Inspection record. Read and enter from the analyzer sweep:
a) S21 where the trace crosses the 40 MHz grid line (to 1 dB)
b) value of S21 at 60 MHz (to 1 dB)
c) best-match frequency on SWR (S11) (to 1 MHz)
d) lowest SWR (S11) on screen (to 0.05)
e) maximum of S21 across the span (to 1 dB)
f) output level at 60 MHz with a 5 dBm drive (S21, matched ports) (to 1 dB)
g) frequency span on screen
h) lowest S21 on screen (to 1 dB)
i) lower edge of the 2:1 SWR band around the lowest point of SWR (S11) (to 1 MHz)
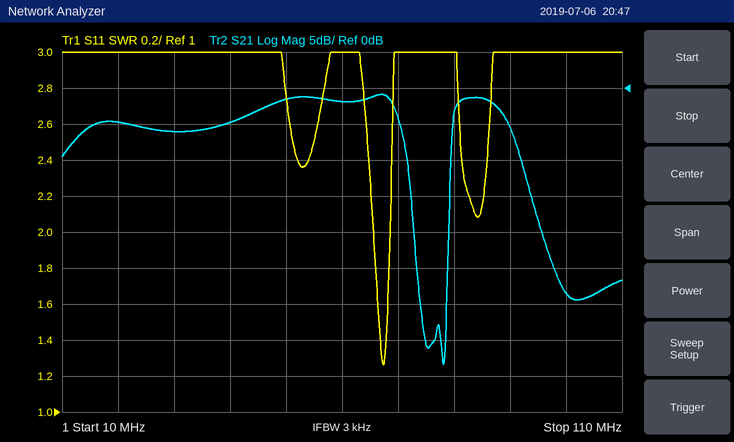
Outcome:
-5 dB
-2 dB
67 MHz
1.25
-1 dB
3 dBm
100 MHz
-38 dB
66 MHz
